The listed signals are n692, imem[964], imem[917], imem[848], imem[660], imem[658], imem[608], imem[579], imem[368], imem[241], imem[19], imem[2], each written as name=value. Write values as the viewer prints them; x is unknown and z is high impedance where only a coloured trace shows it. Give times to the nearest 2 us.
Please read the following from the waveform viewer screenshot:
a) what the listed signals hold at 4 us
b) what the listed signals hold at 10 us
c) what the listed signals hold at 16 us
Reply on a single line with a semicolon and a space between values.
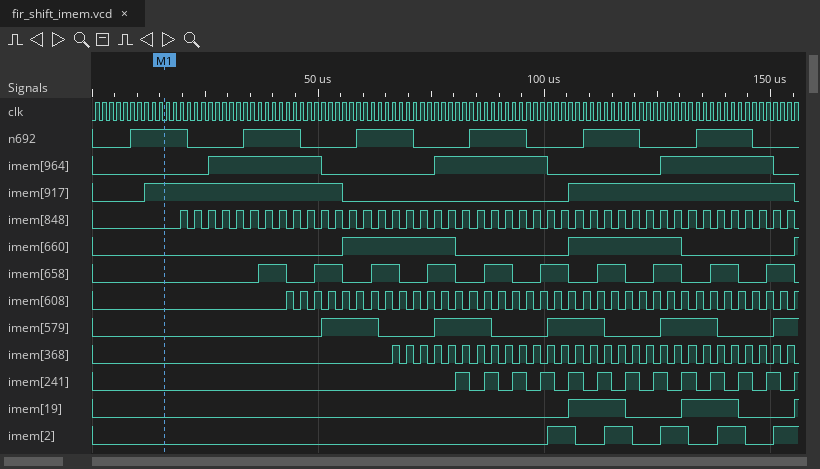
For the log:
n692=0, imem[964]=0, imem[917]=0, imem[848]=0, imem[660]=0, imem[658]=0, imem[608]=0, imem[579]=0, imem[368]=0, imem[241]=0, imem[19]=0, imem[2]=0; n692=1, imem[964]=0, imem[917]=0, imem[848]=0, imem[660]=0, imem[658]=0, imem[608]=0, imem[579]=0, imem[368]=0, imem[241]=0, imem[19]=0, imem[2]=0; n692=1, imem[964]=0, imem[917]=1, imem[848]=0, imem[660]=0, imem[658]=0, imem[608]=0, imem[579]=0, imem[368]=0, imem[241]=0, imem[19]=0, imem[2]=0
